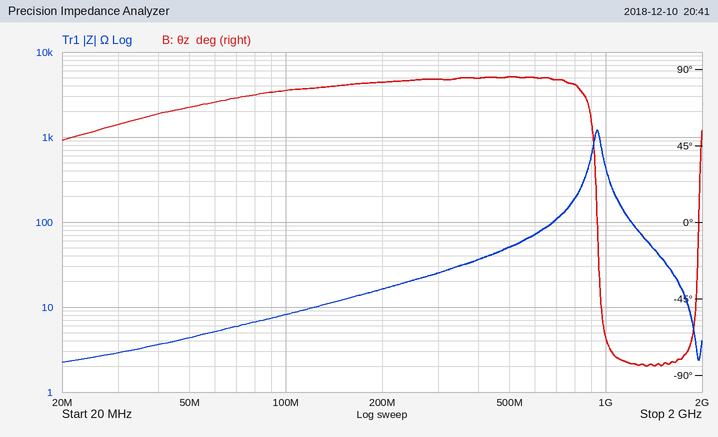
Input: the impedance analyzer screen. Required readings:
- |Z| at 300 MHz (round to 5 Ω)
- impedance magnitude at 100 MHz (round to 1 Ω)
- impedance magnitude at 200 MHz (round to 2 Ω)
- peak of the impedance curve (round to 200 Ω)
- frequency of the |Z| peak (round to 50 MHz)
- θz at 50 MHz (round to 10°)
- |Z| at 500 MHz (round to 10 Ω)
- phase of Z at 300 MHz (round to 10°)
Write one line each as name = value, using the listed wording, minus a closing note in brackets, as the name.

|Z| at 300 MHz = 25 Ω
impedance magnitude at 100 MHz = 8 Ω
impedance magnitude at 200 MHz = 16 Ω
peak of the impedance curve = 1.2 kΩ
frequency of the |Z| peak = 950 MHz
θz at 50 MHz = 70°
|Z| at 500 MHz = 50 Ω
phase of Z at 300 MHz = 80°
